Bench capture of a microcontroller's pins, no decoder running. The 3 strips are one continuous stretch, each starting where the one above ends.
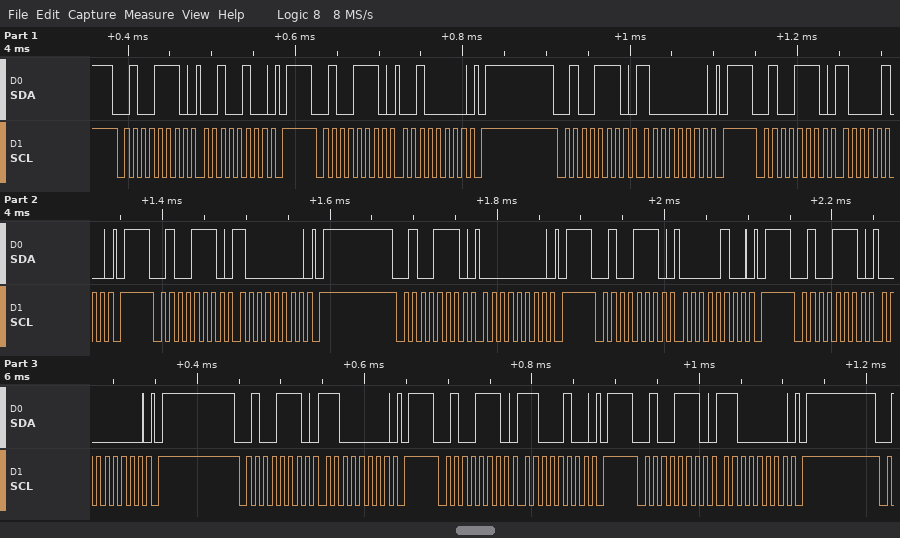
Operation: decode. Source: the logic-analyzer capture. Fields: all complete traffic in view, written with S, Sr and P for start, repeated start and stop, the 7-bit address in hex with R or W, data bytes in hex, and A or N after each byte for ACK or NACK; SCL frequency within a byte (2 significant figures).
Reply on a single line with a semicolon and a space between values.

S 27W A 24 A P S 27W A 20 A P S 27W A 80 A P S 27W A 84 A P S 27W A 80 A P S 27W A 00 A P S 27W A 04 A P S 27W A 00 A P S 27W A C0 A P S 27W A C4 A P S 27W A C0 A P; 100 kHz
